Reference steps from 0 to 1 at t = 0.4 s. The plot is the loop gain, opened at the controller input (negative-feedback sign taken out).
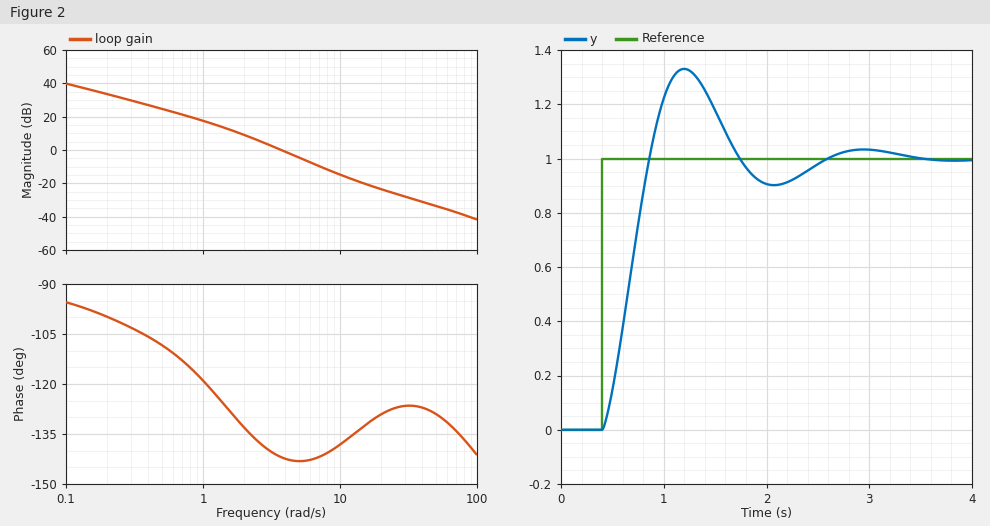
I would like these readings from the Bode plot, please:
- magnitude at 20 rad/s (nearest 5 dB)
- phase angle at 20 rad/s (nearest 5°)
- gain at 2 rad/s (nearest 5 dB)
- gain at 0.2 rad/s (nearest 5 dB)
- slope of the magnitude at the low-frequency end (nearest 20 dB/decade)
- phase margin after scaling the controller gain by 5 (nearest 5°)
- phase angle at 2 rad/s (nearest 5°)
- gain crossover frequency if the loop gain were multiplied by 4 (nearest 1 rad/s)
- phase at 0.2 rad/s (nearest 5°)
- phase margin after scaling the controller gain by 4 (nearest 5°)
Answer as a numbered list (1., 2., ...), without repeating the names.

1. -25 dB
2. -130°
3. 10 dB
4. 35 dB
5. -20 dB/decade
6. 40°
7. -135°
8. 8 rad/s
9. -100°
10. 40°
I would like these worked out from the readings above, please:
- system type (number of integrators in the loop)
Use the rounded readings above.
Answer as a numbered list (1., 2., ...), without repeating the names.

1. 1
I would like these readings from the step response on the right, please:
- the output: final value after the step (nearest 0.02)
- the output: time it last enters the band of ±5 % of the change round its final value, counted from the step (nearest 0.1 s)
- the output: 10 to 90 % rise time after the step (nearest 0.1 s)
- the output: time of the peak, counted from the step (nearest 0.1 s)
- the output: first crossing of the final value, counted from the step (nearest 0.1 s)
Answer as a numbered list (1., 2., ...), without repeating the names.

1. 1.00
2. 2.0 s
3. 0.3 s
4. 0.8 s
5. 0.5 s
